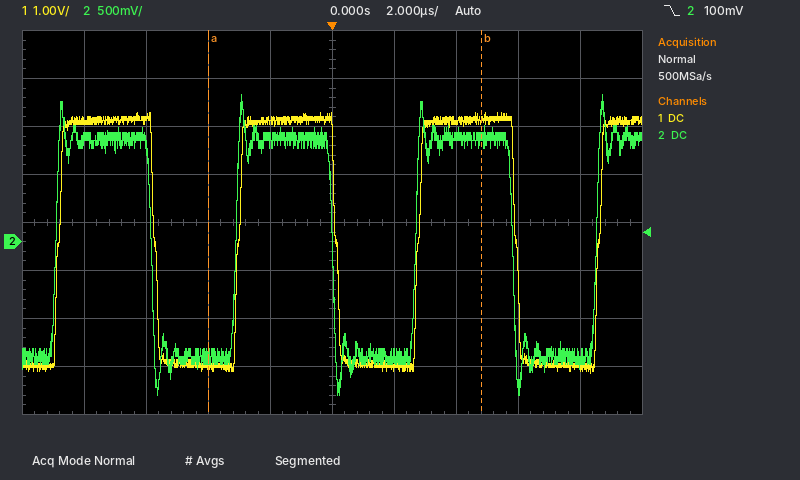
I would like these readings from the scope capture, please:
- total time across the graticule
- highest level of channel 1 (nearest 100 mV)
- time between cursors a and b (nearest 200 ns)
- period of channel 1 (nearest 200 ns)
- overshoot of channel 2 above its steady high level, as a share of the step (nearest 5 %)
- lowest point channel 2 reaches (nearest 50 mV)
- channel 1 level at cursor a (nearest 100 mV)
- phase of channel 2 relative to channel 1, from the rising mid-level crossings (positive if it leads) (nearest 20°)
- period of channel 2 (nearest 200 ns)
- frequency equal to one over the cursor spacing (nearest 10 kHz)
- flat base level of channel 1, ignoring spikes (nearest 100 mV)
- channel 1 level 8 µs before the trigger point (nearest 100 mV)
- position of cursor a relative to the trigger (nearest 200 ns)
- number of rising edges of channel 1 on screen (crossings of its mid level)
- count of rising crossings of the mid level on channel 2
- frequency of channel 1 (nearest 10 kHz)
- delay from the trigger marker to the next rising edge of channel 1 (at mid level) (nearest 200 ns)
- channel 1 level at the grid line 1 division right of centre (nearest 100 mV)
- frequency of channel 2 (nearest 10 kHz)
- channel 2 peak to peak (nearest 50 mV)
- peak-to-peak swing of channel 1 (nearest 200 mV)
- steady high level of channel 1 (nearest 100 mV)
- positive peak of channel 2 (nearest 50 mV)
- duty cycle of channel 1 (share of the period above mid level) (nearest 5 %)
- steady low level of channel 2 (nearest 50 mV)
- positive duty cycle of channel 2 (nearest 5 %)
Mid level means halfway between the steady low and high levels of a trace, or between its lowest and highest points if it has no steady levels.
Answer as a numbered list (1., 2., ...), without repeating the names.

1. 20 µs
2. 2.7 V
3. 8.8 µs
4. 5.8 µs
5. 20 %
6. -1.60 V
7. -2.6 V
8. 0°
9. 5.8 µs
10. 110 kHz
11. -2.6 V
12. 2.5 V
13. -4.0 µs
14. 4
15. 4
16. 170 kHz
17. 2.8 µs
18. -2.6 V
19. 170 kHz
20. 3.15 V
21. 5.4 V
22. 2.5 V
23. 1.55 V
24. 55 %
25. -1.20 V
26. 55 %
